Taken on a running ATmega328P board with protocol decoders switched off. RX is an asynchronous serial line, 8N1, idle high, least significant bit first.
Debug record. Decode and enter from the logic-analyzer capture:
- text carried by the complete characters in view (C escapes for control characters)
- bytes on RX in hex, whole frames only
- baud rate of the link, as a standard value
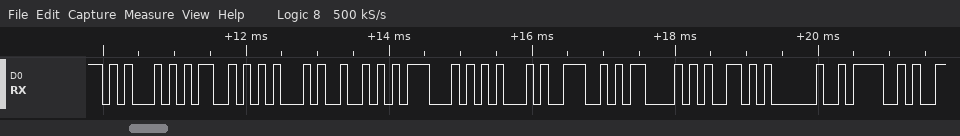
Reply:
"EMERGENCY O"
45 4D 45 52 47 45 4E 43 59 20 4F
9600 baud
